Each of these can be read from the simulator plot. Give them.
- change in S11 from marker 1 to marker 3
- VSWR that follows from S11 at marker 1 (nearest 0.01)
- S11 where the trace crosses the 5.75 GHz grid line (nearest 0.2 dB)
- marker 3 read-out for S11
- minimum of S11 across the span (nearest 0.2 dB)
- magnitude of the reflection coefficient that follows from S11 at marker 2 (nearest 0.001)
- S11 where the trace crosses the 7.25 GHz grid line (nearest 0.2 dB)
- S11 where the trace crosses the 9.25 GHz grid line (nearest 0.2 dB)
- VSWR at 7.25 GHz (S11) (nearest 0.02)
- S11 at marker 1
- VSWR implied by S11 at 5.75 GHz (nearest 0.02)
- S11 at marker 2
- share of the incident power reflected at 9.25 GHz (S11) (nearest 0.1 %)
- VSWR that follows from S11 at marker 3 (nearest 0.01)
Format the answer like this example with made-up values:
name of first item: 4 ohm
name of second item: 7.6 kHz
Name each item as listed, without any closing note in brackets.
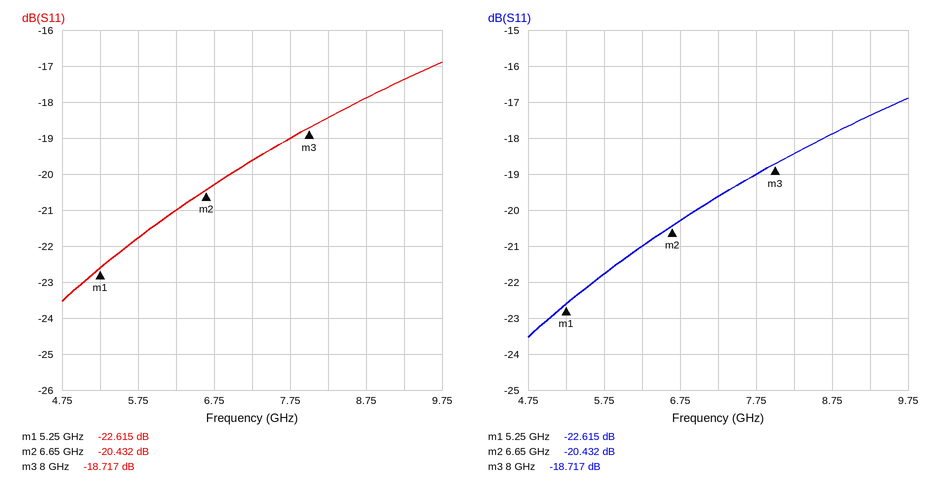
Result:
change in S11 from marker 1 to marker 3: 3.898 dB
VSWR that follows from S11 at marker 1: 1.16
S11 where the trace crosses the 5.75 GHz grid line: -21.8 dB
marker 3 read-out for S11: -18.717 dB
minimum of S11 across the span: -23.6 dB
magnitude of the reflection coefficient that follows from S11 at marker 2: 0.095
S11 where the trace crosses the 7.25 GHz grid line: -19.6 dB
S11 where the trace crosses the 9.25 GHz grid line: -17.4 dB
VSWR at 7.25 GHz (S11): 1.24
S11 at marker 1: -22.615 dB
VSWR implied by S11 at 5.75 GHz: 1.18
S11 at marker 2: -20.432 dB
share of the incident power reflected at 9.25 GHz (S11): 1.8 %
VSWR that follows from S11 at marker 3: 1.26
